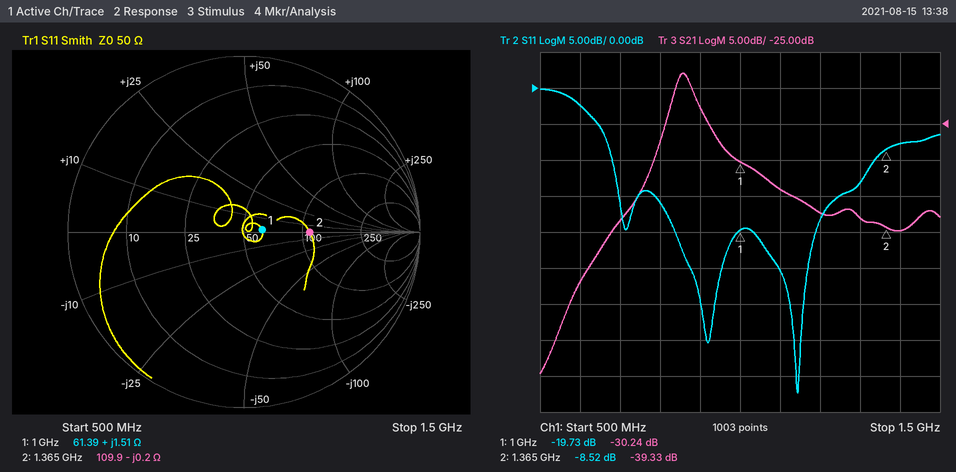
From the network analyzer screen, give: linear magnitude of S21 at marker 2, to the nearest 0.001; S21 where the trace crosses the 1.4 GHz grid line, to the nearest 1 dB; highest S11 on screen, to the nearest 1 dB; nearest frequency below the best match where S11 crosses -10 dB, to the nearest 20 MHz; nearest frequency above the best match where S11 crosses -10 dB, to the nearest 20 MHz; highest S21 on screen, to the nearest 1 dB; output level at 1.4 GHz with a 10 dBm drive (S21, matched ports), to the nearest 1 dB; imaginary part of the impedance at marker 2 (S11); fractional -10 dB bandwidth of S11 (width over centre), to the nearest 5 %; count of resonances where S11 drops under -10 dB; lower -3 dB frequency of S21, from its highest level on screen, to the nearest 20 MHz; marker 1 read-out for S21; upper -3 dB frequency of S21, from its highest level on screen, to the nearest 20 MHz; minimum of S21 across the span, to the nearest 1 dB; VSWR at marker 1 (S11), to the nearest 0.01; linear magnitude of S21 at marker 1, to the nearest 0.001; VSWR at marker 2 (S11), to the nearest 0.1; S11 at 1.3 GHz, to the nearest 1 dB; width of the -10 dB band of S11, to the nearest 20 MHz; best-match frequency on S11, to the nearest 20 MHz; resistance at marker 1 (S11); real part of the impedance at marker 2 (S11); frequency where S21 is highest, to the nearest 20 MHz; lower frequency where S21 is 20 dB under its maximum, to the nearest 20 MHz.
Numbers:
0.011
-40 dB
0 dB
680 MHz
1.34 GHz
-18 dB
-30 dBm
-0.2 Ω
65 %
3
840 MHz
-30.24 dB
880 MHz
-60 dB
1.23
0.031
2.2
-13 dB
660 MHz
1.14 GHz
61.39 Ω
109.9 Ω
860 MHz
700 MHz
